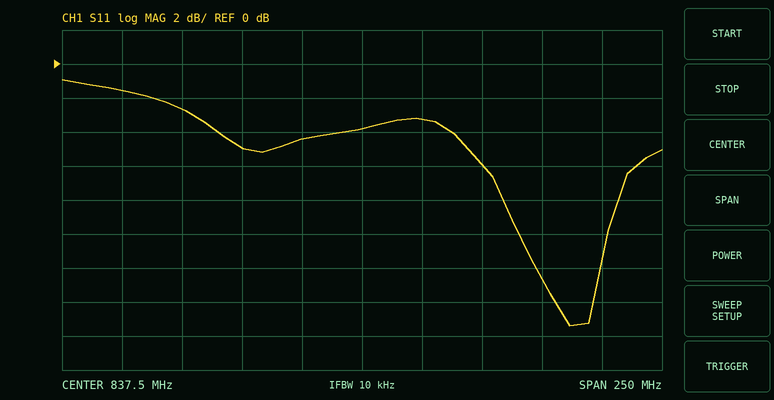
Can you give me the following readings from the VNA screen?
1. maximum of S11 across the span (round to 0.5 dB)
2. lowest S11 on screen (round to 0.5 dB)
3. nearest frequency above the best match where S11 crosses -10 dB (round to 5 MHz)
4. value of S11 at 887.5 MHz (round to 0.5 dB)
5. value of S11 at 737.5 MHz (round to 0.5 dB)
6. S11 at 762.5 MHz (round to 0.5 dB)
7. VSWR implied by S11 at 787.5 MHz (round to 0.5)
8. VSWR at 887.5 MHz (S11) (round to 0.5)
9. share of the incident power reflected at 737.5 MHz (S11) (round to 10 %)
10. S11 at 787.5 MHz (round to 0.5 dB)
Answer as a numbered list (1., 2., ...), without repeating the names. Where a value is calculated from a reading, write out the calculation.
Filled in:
1. -1.0 dB
2. -15.5 dB
3. 940 MHz
4. -6.0 dB
5. -1.5 dB
6. -2.5 dB
7. |Γ| = 10^(-5/20) = 0.5623; VSWR = (1 + 0.5623)/(1 − 0.5623) ≈ 3.57, so 3.5 to the nearest 0.5
8. |Γ| = 10^(-6/20) = 0.5012; VSWR = (1 + 0.5012)/(1 − 0.5012) ≈ 3.0
9. 10^(-1.5/10) ≈ 70.8 %, so 70 % to the nearest 10 %
10. -5.0 dB
